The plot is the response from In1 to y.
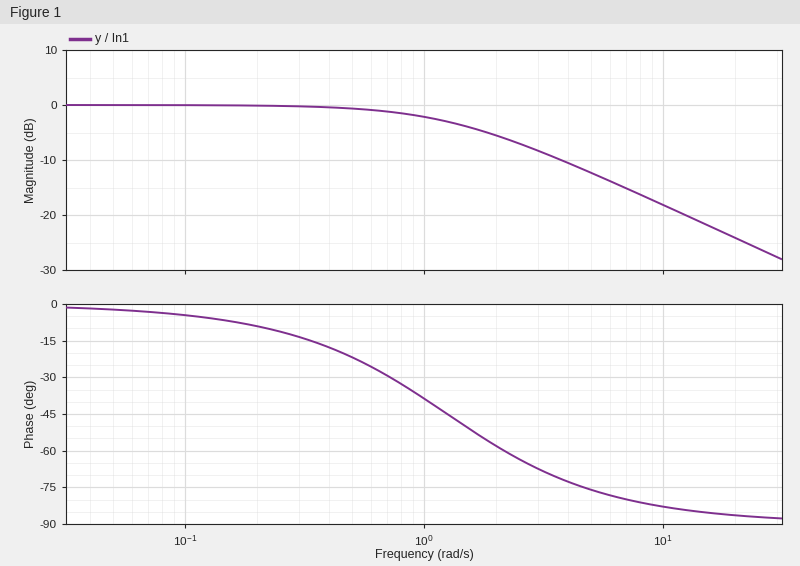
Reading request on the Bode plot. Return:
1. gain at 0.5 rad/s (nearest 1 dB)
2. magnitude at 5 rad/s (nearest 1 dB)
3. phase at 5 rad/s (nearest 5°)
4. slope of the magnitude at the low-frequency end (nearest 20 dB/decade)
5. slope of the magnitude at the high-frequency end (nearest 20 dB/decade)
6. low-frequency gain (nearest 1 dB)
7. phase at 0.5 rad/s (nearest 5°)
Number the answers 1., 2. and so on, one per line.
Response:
1. -1 dB
2. -12 dB
3. -75°
4. 0 dB/decade
5. -20 dB/decade
6. 0 dB
7. -20°
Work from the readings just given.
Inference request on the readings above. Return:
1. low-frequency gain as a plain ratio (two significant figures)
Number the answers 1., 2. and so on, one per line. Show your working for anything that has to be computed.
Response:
1. 10^(0 / 20) = 1.0
